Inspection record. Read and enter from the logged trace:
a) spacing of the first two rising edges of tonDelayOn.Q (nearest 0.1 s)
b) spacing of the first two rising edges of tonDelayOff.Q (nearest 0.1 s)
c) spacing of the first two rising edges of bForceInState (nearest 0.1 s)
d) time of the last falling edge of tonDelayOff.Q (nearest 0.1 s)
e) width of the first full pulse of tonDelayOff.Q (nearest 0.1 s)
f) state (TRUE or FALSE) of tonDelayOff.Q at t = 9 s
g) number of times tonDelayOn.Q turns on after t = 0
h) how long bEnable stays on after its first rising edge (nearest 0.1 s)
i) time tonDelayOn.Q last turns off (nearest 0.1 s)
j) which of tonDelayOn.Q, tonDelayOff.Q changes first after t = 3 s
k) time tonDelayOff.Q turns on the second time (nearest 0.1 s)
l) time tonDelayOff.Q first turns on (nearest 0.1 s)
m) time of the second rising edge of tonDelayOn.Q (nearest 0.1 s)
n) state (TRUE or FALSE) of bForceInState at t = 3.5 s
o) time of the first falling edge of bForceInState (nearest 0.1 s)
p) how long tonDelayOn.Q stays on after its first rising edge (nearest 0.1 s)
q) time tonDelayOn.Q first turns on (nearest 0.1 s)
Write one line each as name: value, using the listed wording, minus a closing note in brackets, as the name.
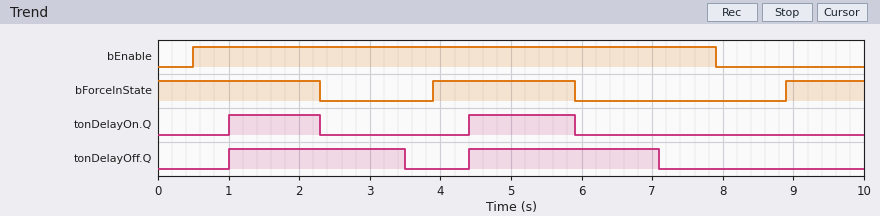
spacing of the first two rising edges of tonDelayOn.Q: 3.4 s
spacing of the first two rising edges of tonDelayOff.Q: 3.4 s
spacing of the first two rising edges of bForceInState: 5.0 s
time of the last falling edge of tonDelayOff.Q: 7.1 s
width of the first full pulse of tonDelayOff.Q: 2.5 s
state (TRUE or FALSE) of tonDelayOff.Q at t = 9 s: FALSE
number of times tonDelayOn.Q turns on after t = 0: 2
how long bEnable stays on after its first rising edge: 7.4 s
time tonDelayOn.Q last turns off: 5.9 s
which of tonDelayOn.Q, tonDelayOff.Q changes first after t = 3 s: tonDelayOff.Q
time tonDelayOff.Q turns on the second time: 4.4 s
time tonDelayOff.Q first turns on: 1.0 s
time of the second rising edge of tonDelayOn.Q: 4.4 s
state (TRUE or FALSE) of bForceInState at t = 3.5 s: FALSE
time of the first falling edge of bForceInState: 2.3 s
how long tonDelayOn.Q stays on after its first rising edge: 1.3 s
time tonDelayOn.Q first turns on: 1.0 s
